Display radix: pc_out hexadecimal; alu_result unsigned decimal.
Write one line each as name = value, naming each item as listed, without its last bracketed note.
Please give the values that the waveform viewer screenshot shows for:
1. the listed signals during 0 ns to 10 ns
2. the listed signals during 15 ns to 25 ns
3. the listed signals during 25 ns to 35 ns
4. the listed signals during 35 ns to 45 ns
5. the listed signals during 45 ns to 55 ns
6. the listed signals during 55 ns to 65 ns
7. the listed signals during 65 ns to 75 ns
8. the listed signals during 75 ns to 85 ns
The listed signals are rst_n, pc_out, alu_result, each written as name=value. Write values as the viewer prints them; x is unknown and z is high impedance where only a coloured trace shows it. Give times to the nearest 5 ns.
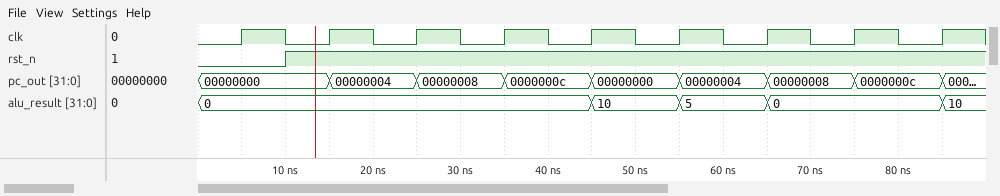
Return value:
the listed signals during 0 ns to 10 ns = rst_n=0, pc_out=00000000, alu_result=0
the listed signals during 15 ns to 25 ns = rst_n=1, pc_out=00000004, alu_result=0
the listed signals during 25 ns to 35 ns = rst_n=1, pc_out=00000008, alu_result=0
the listed signals during 35 ns to 45 ns = rst_n=1, pc_out=0000000c, alu_result=0
the listed signals during 45 ns to 55 ns = rst_n=1, pc_out=00000000, alu_result=10
the listed signals during 55 ns to 65 ns = rst_n=1, pc_out=00000004, alu_result=5
the listed signals during 65 ns to 75 ns = rst_n=1, pc_out=00000008, alu_result=0
the listed signals during 75 ns to 85 ns = rst_n=1, pc_out=0000000c, alu_result=0
